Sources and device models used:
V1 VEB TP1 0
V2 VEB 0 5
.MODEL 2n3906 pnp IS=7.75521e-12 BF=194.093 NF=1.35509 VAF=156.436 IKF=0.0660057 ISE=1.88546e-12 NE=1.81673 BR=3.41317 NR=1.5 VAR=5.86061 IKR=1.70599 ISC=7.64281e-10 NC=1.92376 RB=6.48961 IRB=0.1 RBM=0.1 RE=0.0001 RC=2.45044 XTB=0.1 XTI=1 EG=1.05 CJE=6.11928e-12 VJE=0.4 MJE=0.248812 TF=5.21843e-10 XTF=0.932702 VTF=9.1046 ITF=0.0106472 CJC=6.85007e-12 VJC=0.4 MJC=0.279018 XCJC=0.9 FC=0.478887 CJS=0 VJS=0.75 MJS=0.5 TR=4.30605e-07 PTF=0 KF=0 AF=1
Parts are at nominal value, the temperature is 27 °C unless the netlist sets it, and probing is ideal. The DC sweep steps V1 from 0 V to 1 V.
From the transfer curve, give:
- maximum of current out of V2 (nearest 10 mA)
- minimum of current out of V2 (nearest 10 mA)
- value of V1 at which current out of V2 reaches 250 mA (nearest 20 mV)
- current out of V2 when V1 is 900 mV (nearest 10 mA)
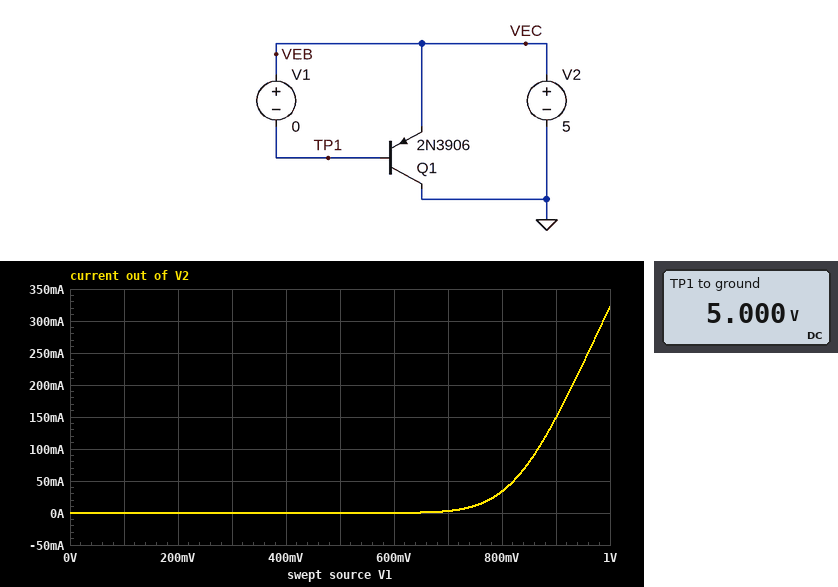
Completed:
320 mA
0 A
960 mV
150 mA
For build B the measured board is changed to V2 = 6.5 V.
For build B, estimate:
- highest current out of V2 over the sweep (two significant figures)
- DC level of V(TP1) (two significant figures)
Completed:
330 mA
6.5 V
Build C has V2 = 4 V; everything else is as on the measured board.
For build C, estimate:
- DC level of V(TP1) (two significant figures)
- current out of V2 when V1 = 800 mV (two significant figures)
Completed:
4.0 V
33 mA
